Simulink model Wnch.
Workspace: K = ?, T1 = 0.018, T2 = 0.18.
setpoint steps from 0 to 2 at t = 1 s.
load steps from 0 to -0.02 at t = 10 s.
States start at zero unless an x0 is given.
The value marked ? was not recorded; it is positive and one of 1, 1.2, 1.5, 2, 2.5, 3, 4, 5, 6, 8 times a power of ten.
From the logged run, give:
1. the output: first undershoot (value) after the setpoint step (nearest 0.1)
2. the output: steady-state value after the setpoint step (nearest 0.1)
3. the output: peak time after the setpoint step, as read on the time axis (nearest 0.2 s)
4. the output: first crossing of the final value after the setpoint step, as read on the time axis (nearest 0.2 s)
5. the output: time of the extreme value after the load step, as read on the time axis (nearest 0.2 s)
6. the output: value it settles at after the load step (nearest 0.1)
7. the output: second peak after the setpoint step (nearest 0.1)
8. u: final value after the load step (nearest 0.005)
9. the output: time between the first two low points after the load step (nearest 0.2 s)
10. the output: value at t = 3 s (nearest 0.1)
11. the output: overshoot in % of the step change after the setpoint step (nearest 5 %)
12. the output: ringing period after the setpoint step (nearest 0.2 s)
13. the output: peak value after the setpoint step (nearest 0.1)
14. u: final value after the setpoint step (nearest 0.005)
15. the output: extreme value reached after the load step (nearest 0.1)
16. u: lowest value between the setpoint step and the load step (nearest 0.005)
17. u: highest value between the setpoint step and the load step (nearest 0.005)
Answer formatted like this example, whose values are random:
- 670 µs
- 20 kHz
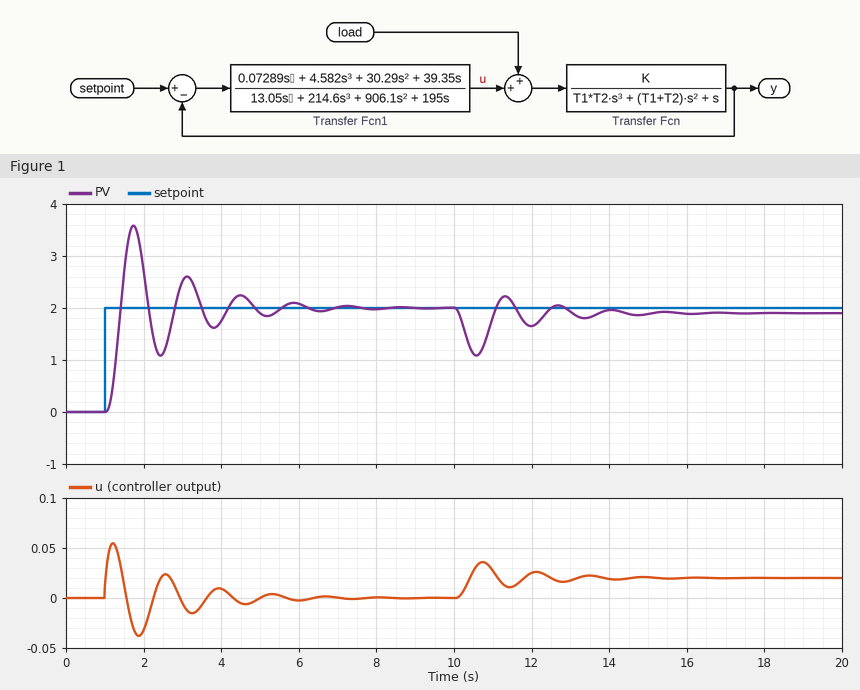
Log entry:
- 1.1
- 2.0
- 1.8 s
- 1.4 s
- 10.6 s
- 1.9
- 2.6
- 0.020
- 1.4 s
- 2.5
- 80 %
- 1.4 s
- 3.6
- 0.000
- 1.1
- -0.040
- 0.055
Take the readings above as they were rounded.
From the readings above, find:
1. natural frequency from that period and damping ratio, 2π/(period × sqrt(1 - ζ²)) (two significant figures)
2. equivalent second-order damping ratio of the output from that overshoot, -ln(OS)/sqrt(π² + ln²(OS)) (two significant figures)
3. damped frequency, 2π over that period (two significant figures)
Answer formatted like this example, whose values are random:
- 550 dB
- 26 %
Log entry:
- 4.5 rad/s
- 0.071
- 4.5 rad/s
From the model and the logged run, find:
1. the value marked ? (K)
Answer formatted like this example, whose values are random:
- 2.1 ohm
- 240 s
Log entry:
- 200
